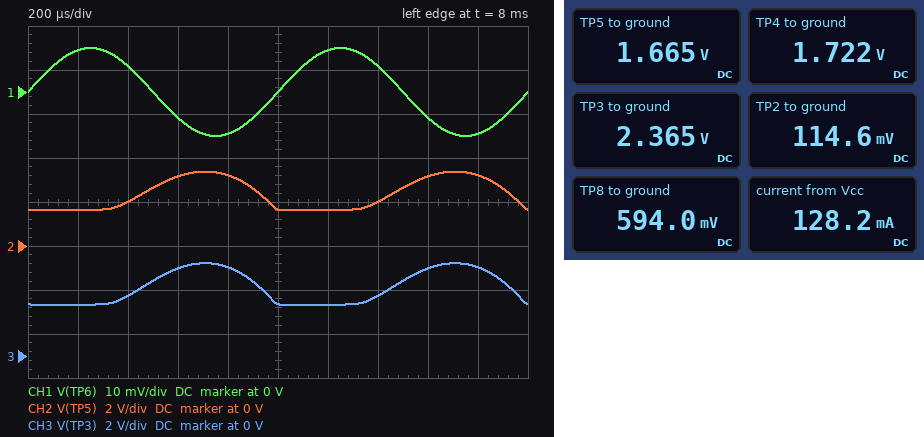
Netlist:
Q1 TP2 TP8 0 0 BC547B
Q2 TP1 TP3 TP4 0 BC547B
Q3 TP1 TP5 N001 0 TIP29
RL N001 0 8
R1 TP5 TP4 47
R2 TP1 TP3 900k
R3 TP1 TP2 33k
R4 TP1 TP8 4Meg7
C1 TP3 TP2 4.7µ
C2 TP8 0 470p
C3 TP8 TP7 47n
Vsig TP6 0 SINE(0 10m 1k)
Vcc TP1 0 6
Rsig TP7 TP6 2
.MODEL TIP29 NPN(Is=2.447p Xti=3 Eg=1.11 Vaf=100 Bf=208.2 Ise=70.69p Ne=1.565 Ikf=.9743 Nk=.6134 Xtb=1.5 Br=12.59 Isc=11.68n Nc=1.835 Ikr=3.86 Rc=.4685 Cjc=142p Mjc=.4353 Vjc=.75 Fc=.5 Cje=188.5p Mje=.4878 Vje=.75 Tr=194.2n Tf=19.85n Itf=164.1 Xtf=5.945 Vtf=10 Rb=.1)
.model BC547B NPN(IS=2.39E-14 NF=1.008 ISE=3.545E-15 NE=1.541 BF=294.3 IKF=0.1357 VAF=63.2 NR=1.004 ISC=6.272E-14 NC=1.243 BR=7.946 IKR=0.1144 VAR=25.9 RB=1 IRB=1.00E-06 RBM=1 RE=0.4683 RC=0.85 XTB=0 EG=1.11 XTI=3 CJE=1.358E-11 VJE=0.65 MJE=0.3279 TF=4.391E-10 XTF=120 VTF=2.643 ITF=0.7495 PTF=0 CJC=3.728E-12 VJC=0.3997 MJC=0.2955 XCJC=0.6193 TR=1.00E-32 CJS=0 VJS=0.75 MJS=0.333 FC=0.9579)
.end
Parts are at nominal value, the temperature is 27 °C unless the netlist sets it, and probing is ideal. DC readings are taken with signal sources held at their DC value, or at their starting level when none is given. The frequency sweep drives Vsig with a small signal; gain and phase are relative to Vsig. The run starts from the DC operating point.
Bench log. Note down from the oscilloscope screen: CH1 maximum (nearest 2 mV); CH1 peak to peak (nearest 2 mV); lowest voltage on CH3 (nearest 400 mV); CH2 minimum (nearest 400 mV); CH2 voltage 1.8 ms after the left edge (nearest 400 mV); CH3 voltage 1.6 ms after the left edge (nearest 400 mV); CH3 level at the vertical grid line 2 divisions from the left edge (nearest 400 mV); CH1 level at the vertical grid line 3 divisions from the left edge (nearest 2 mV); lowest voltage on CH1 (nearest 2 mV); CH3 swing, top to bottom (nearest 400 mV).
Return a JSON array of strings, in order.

["10 mV", "20 mV", "2.4 V", "1.6 V", "3.2 V", "4.0 V", "2.8 V", "-6 mV", "-10 mV", "2.0 V"]
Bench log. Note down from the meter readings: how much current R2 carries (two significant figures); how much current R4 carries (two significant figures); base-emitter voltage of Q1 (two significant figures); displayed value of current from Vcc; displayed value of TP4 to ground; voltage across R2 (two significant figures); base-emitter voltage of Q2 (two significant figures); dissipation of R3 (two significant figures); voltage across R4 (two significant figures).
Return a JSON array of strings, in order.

["4.0 µA", "1.2 µA", "590 mV", "128.2 mA", "1.722 V", "3.6 V", "640 mV", "1.0 mW", "5.4 V"]
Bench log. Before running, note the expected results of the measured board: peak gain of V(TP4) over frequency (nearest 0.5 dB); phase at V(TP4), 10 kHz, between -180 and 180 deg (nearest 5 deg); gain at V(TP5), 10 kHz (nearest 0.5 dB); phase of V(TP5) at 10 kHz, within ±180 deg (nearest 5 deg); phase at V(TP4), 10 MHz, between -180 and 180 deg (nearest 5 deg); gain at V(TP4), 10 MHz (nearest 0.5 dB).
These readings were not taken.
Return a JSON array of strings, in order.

["32.5 dB", "-165 deg", "32.0 dB", "-165 deg", "75 deg", "4.5 dB"]
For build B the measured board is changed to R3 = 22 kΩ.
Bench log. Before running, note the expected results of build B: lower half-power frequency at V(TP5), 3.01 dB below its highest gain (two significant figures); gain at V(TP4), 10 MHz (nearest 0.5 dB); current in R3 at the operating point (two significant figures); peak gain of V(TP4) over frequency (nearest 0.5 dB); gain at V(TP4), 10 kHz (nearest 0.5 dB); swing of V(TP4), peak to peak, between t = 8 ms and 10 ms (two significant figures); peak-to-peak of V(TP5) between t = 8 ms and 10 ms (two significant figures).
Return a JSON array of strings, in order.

["2.5 kHz", "8.5 dB", "270 µA", "40.0 dB", "39.5 dB", "2.2 V", "2.1 V"]
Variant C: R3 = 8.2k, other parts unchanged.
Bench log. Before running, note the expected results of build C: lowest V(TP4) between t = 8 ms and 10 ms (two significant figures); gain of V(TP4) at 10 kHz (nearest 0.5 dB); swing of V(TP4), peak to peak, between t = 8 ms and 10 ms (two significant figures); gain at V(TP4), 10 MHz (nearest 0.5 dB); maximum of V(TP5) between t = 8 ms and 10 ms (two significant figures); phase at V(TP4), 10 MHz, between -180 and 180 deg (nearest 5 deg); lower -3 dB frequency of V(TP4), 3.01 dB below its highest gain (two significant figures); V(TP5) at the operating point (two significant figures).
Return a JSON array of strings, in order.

["760 mV", "39.5 dB", "1.8 V", "16.0 dB", "2.5 V", "90 deg", "150 Hz", "1.7 V"]
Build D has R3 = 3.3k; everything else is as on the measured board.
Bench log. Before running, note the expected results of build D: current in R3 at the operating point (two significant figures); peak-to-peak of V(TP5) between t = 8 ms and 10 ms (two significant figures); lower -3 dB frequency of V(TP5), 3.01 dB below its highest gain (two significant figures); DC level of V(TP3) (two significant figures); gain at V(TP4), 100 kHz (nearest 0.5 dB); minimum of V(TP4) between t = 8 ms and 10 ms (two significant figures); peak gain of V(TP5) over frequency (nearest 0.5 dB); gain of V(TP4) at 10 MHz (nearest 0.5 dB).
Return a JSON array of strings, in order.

["350 µA", "750 mV", "150 Hz", "2.4 V", "32.0 dB", "1.3 V", "31.5 dB", "16.0 dB"]
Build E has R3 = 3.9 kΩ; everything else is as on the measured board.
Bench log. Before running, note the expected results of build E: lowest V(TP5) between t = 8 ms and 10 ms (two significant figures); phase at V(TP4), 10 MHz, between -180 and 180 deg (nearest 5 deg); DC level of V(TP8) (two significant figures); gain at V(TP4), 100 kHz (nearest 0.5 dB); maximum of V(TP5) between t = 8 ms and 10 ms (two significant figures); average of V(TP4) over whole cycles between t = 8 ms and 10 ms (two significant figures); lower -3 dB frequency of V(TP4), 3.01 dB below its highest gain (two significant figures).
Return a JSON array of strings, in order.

["1.2 V", "95 deg", "610 mV", "33.5 dB", "2.1 V", "1.7 V", "150 Hz"]
